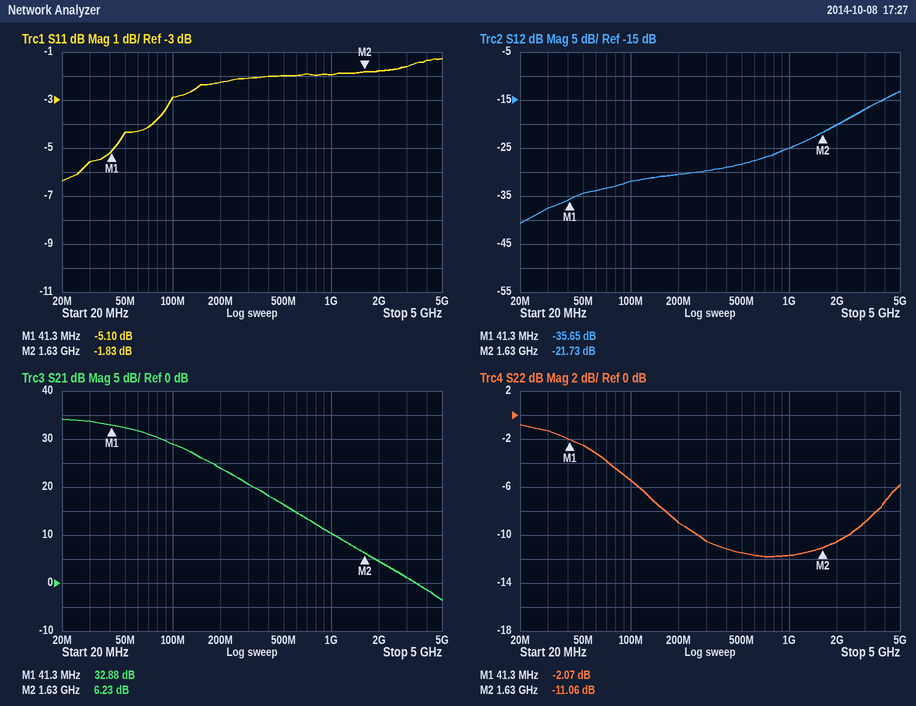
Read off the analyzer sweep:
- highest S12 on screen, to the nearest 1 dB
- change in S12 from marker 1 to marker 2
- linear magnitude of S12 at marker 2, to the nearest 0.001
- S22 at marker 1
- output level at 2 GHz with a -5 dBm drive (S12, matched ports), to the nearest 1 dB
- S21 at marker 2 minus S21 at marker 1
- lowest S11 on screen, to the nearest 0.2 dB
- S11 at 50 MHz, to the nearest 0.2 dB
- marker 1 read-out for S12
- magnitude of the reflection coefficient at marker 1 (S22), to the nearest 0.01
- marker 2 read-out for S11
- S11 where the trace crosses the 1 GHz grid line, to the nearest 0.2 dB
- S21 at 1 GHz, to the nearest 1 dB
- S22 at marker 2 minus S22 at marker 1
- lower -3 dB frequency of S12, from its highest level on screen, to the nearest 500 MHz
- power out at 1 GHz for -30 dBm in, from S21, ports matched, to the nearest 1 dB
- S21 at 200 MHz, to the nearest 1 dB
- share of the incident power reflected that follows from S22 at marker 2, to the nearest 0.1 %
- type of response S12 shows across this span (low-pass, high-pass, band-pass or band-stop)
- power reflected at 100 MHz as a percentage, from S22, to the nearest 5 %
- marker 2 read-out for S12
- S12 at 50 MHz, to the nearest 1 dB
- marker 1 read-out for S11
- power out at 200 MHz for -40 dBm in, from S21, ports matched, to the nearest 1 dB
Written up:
-13 dB
13.92 dB
0.082
-2.07 dB
-25 dBm
-26.65 dB
-6.4 dB
-4.4 dB
-35.65 dB
0.79
-1.83 dB
-2.0 dB
10 dB
-8.99 dB
3.5 GHz
-20 dBm
24 dB
7.8 %
high-pass
30 %
-21.73 dB
-34 dB
-5.10 dB
-16 dBm
